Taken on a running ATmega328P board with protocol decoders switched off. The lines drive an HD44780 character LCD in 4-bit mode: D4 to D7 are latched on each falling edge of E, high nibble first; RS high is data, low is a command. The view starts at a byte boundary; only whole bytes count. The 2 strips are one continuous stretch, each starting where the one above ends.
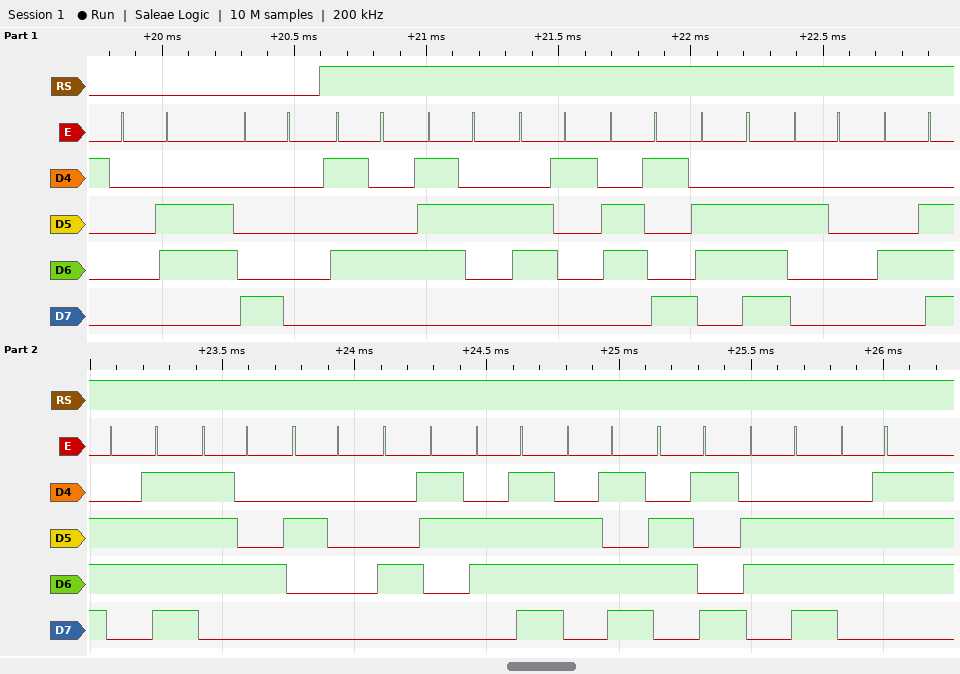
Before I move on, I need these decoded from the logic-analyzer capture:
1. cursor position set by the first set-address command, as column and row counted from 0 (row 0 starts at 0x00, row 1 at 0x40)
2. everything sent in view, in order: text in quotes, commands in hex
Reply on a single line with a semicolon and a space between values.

column 0, row 0; 0x06 0x80 "Train Not Coming"
